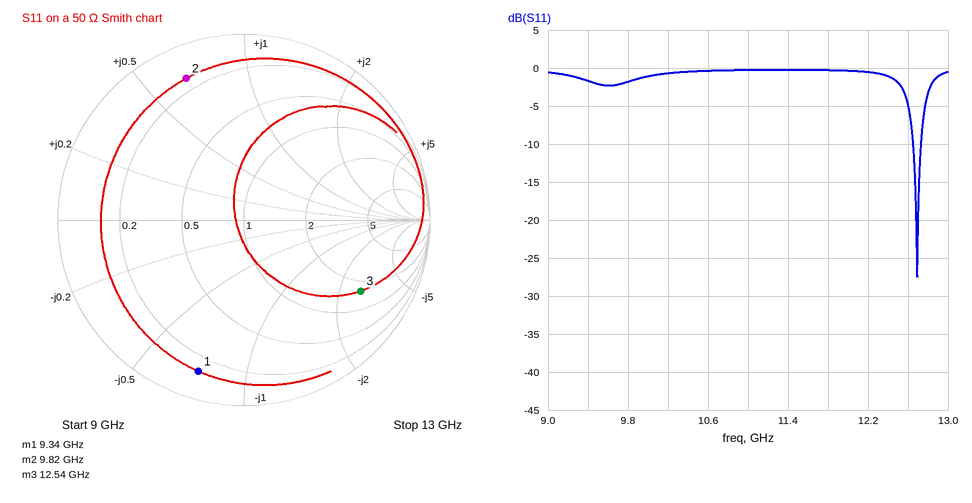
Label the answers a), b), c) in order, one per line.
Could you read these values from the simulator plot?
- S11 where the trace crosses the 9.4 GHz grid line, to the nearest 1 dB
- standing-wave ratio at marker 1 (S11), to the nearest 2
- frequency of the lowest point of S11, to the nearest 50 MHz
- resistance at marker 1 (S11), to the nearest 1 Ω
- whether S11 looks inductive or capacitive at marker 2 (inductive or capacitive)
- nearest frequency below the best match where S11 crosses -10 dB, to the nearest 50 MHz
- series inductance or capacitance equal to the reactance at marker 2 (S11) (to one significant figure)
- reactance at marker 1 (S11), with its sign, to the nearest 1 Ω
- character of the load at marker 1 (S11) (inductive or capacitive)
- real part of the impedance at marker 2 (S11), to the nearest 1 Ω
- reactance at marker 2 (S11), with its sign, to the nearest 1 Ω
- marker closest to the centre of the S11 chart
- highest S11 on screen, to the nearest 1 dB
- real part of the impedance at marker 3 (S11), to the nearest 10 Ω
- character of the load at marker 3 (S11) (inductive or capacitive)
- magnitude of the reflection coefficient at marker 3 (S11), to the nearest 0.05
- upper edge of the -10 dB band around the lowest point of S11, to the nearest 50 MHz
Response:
a) -2 dB
b) 12
c) 12.70 GHz
d) 6 Ω
e) inductive
f) 12.65 GHz
g) 500 pH
h) -37 Ω
i) capacitive
j) 7 Ω
k) +33 Ω
l) marker 3
m) 0 dB
n) 80 Ω
o) capacitive
p) 0.75
q) 12.75 GHz
